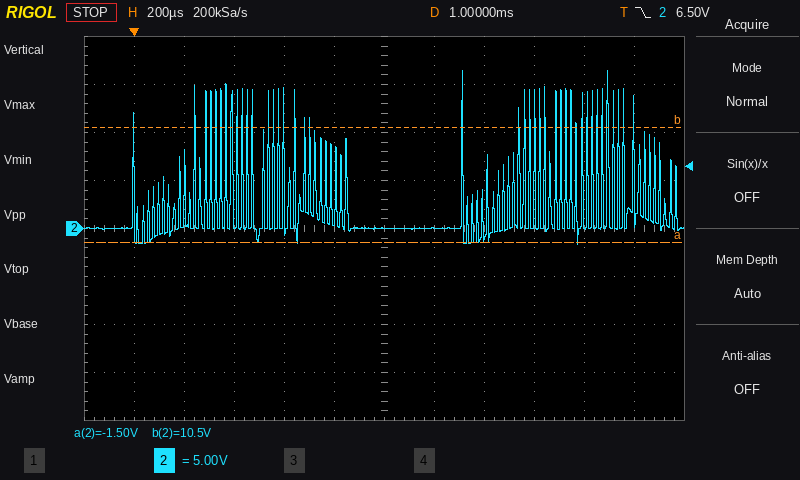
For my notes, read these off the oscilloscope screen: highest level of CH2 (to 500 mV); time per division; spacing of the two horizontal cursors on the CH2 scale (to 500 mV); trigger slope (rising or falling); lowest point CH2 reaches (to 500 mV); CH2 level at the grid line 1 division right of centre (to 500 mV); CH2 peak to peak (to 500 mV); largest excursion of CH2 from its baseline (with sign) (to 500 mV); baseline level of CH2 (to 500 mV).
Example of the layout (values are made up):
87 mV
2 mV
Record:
16.5 V
200 µs
12.0 V
falling
-1.5 V
0.0 V
18.0 V
+16.5 V
0.0 V
